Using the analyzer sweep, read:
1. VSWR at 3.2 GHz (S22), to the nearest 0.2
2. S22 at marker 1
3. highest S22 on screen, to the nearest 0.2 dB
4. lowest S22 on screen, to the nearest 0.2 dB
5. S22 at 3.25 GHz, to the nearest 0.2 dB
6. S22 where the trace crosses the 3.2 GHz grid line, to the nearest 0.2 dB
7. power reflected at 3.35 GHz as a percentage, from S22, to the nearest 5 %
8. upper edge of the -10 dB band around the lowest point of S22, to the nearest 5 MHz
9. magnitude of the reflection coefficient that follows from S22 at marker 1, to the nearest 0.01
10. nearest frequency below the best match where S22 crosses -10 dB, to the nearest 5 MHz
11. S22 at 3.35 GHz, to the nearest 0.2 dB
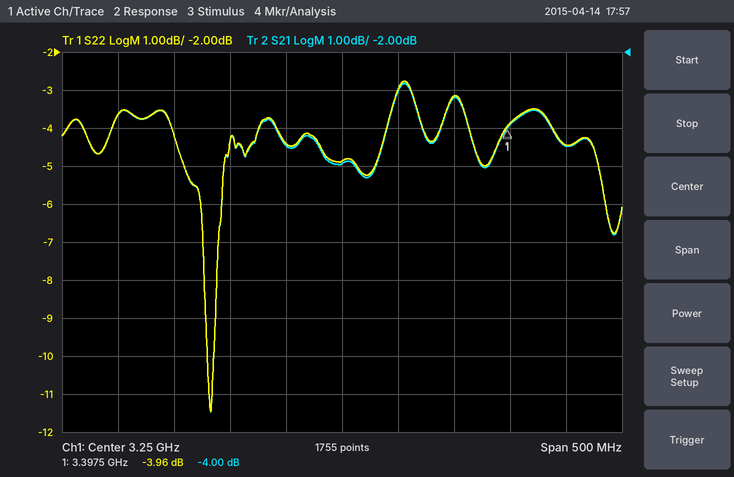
4.0
-3.96 dB
-2.8 dB
-11.4 dB
-4.8 dB
-4.4 dB
50 %
3.135 GHz
0.63
3.130 GHz
-3.2 dB
